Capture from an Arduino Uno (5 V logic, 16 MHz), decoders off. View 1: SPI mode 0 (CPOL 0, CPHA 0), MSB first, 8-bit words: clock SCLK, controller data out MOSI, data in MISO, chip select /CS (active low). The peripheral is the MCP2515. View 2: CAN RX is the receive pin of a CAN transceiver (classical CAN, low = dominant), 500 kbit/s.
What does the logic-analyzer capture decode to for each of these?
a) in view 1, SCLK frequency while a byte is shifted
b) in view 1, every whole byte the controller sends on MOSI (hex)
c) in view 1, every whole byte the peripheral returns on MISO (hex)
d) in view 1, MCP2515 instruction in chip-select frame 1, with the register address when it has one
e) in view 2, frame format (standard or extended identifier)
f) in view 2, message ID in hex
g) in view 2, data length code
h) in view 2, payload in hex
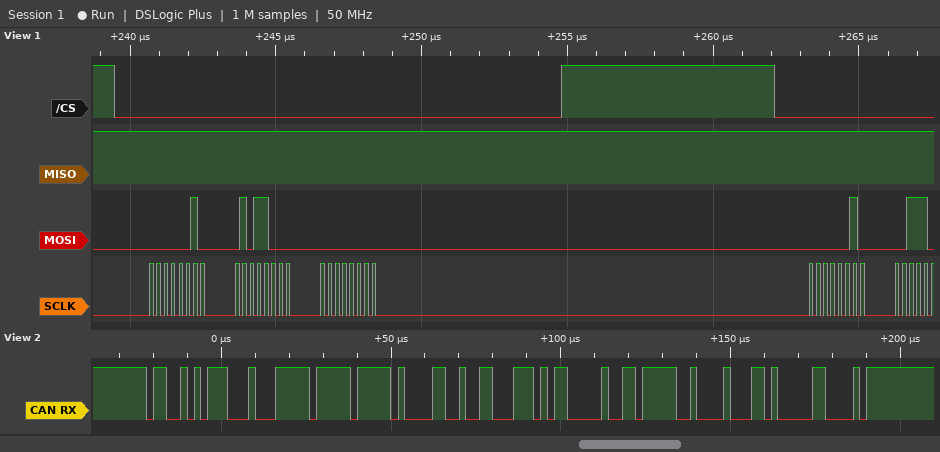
4 MHz
02 58 00 02
FF FF FF FF
WRITE 0x58
standard
0x657
8
FF FF 0C 98 EB 01 BE 84
